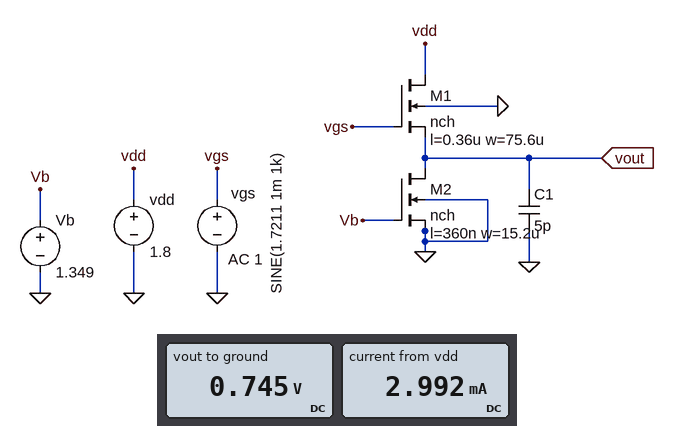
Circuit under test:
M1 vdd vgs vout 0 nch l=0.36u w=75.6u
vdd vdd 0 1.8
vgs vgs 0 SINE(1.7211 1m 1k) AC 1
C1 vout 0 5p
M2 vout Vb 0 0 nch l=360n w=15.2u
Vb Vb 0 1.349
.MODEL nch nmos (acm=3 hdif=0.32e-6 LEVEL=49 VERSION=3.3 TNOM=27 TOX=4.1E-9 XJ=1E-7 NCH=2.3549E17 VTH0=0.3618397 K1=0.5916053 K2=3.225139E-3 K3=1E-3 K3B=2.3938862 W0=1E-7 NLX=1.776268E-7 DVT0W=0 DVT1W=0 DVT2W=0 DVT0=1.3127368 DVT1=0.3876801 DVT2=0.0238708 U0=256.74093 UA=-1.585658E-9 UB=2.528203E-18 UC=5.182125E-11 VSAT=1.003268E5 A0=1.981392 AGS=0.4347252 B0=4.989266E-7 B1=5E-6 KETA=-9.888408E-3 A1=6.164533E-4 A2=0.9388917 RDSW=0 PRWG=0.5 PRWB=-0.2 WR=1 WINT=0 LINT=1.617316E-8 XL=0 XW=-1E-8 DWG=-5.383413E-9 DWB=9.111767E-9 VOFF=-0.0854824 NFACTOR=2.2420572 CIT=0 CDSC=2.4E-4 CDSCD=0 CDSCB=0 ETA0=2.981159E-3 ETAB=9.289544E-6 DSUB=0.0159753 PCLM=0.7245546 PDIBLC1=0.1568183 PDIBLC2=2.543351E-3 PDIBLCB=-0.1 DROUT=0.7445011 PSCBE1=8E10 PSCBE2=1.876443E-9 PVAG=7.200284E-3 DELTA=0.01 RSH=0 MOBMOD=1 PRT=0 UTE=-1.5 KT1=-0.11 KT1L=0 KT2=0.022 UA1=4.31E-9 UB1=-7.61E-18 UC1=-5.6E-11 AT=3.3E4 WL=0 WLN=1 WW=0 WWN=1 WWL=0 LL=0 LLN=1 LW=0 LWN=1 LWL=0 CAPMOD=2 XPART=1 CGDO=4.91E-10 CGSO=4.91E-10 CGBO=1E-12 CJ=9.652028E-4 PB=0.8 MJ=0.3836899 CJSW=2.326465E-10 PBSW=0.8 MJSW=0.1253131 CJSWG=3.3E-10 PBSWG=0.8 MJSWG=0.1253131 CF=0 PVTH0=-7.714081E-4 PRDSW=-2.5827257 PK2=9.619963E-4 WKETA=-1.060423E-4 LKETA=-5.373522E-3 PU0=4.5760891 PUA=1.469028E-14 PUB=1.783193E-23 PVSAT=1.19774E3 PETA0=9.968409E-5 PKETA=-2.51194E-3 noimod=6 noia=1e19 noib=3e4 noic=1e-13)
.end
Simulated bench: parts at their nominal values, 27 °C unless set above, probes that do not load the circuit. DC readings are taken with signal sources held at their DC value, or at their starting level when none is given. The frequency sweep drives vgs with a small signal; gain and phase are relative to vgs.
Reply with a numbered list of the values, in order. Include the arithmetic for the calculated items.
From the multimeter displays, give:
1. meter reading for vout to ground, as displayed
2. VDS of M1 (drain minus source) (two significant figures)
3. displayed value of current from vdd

1. 0.745 V
2. 1.8 V - 745 mV = 1.1 V
3. 2.992 mA
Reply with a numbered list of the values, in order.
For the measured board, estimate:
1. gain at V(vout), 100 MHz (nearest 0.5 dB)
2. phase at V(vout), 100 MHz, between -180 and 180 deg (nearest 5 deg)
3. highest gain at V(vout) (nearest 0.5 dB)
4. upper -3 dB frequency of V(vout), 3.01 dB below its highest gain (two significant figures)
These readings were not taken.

1. -2.0 dB
2. -10 deg
3. -2.0 dB
4. 600 MHz
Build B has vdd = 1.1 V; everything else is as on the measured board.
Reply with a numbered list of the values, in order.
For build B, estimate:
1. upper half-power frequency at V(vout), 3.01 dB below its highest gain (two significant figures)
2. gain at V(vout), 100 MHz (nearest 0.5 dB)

1. 590 MHz
2. -2.5 dB
